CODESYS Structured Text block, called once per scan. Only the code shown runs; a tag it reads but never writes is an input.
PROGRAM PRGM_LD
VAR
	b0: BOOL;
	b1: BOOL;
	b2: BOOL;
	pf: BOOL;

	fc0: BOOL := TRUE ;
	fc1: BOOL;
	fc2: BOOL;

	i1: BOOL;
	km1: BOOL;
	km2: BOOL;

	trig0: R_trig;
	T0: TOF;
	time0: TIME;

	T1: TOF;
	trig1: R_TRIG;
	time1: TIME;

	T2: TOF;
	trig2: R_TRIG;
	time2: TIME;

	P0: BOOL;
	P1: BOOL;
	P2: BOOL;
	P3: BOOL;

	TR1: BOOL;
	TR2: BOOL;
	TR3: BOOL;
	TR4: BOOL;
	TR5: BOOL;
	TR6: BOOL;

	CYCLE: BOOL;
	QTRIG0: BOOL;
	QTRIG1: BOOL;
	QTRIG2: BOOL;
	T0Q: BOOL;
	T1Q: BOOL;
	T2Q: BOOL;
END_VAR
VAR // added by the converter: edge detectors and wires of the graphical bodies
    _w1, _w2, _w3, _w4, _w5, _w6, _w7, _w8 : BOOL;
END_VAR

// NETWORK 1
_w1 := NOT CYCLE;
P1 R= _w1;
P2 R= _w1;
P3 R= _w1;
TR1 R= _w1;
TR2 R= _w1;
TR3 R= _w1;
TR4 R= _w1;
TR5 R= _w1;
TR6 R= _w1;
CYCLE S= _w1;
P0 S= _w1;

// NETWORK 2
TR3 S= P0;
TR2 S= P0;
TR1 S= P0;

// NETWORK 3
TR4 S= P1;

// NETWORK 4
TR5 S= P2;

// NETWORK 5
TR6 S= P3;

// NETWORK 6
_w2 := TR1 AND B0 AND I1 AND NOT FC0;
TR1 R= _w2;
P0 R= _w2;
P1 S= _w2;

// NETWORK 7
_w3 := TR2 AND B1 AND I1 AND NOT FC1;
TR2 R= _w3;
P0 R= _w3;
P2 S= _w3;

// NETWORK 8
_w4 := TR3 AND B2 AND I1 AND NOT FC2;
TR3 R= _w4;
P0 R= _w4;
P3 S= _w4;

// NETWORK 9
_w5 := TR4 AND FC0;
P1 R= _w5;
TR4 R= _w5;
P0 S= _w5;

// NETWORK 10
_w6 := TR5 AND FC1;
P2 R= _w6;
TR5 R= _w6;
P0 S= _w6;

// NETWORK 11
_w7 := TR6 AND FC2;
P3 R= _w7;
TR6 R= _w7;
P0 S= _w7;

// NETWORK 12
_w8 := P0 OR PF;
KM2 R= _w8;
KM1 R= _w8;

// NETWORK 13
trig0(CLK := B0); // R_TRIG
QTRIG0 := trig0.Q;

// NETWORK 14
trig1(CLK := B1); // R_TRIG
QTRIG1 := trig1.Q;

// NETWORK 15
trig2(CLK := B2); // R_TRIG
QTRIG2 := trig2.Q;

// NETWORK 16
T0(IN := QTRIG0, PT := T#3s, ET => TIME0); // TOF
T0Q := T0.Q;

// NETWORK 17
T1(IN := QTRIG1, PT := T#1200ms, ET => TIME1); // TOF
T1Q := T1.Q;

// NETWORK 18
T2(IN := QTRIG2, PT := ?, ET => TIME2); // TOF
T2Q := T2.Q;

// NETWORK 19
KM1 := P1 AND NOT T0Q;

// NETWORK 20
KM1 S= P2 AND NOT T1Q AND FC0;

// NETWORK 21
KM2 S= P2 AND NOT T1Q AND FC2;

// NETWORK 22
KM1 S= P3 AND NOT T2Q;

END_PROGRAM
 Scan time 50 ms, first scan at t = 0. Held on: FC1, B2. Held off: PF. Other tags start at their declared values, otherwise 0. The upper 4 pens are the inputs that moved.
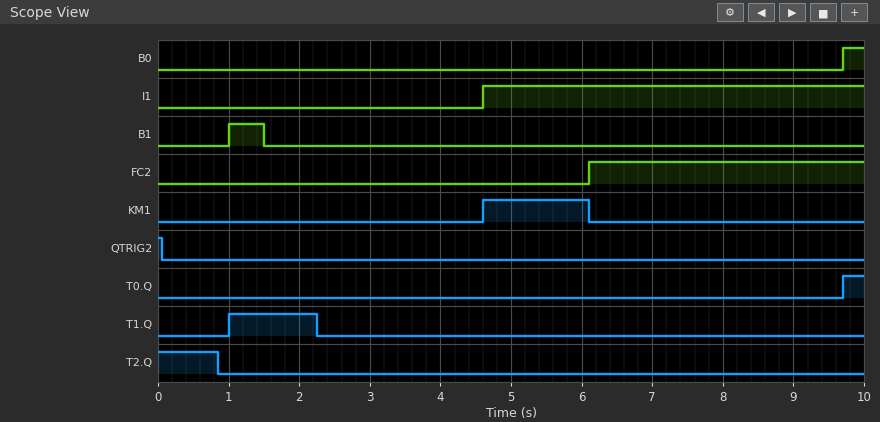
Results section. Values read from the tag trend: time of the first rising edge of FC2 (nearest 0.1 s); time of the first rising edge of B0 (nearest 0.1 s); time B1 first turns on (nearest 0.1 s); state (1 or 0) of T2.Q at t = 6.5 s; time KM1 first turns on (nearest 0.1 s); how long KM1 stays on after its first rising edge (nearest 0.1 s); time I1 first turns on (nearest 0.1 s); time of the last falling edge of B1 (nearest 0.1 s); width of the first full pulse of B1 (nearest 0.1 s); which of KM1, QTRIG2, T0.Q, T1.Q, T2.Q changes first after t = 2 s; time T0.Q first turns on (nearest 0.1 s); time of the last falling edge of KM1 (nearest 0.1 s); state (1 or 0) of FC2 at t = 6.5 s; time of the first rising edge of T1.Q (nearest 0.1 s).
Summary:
6.1 s
9.7 s
1.0 s
0
4.6 s
1.5 s
4.6 s
1.5 s
0.5 s
T1.Q
9.7 s
6.1 s
1
1.0 s
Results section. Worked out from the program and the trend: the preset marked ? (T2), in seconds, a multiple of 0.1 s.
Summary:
0.8 s
